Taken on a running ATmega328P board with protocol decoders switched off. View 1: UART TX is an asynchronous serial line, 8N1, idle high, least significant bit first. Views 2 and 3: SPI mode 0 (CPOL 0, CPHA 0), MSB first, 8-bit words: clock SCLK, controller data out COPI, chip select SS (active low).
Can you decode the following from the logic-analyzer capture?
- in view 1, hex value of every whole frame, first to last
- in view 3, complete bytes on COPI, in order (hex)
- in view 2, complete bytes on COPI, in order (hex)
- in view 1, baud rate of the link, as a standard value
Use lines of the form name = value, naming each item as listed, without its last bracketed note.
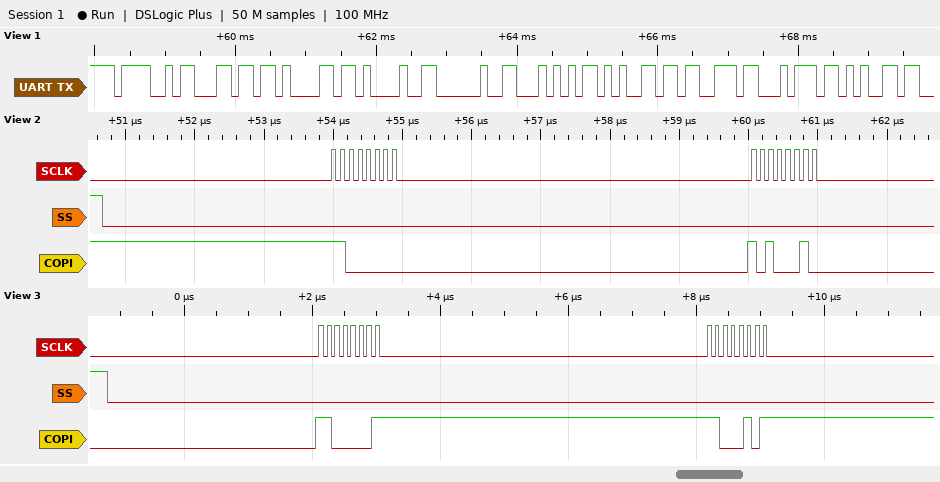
in view 1, hex value of every whole frame, first to last = 4F 6C 61 21 20 54 65 73 74 65
in view 3, complete bytes on COPI, in order = 0xC1 0xC5
in view 2, complete bytes on COPI, in order = C0 A2
in view 1, baud rate of the link, as a standard value = 9600 baud
